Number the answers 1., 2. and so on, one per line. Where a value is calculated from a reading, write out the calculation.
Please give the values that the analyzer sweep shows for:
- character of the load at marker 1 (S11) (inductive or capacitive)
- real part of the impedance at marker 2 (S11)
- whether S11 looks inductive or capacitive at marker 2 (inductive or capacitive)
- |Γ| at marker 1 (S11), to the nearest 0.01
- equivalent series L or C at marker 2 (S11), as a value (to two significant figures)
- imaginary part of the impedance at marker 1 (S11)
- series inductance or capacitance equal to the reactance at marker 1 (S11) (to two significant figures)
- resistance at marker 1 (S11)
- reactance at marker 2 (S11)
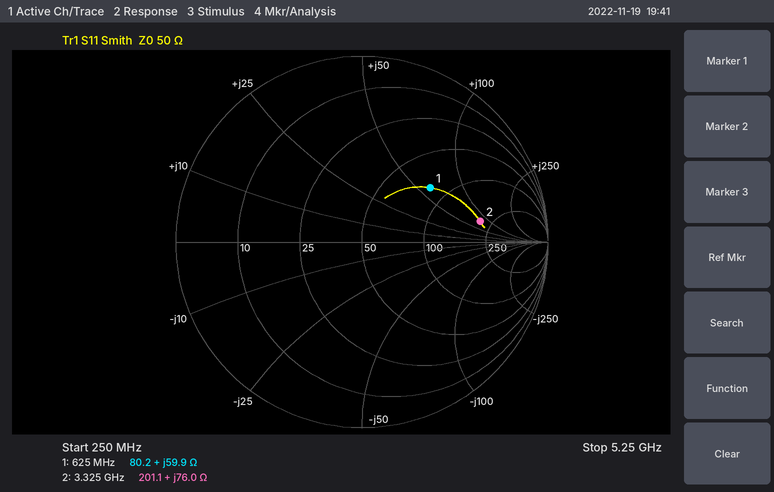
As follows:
1. inductive
2. 201.1 Ω
3. inductive
4. 0.47
5. L = 76 Ω/(2π × 3.325 GHz) ≈ 3.6 nH
6. +59.9 Ω
7. L = 59.9 Ω/(2π × 625 MHz) ≈ 15 nH
8. 80.2 Ω
9. +76.0 Ω
